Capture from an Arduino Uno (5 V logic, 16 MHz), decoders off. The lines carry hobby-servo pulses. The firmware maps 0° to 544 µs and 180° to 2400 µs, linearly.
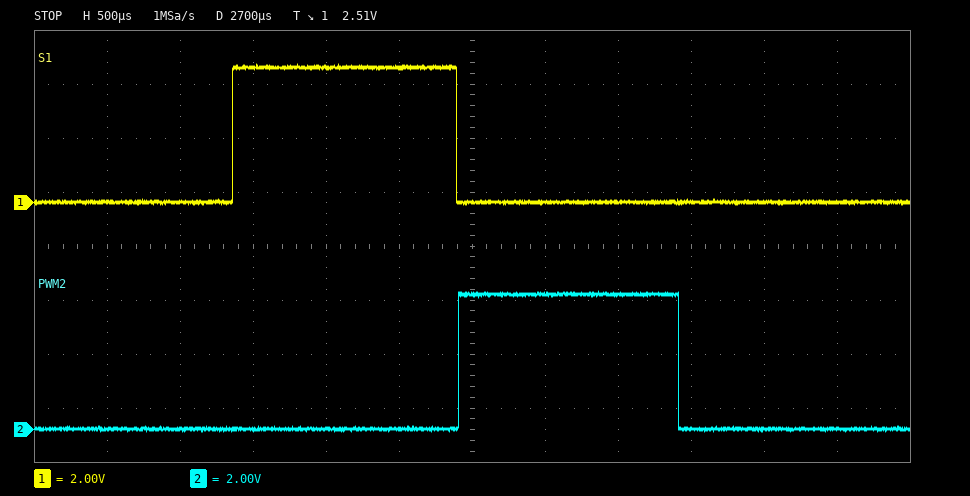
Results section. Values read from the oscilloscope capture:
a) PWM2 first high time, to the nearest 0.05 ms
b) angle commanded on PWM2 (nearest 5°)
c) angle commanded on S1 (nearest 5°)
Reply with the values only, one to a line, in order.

1.50 ms
95°
95°
